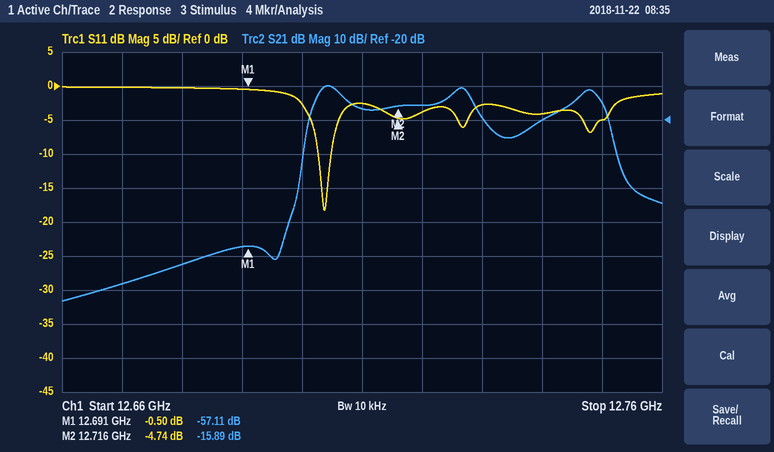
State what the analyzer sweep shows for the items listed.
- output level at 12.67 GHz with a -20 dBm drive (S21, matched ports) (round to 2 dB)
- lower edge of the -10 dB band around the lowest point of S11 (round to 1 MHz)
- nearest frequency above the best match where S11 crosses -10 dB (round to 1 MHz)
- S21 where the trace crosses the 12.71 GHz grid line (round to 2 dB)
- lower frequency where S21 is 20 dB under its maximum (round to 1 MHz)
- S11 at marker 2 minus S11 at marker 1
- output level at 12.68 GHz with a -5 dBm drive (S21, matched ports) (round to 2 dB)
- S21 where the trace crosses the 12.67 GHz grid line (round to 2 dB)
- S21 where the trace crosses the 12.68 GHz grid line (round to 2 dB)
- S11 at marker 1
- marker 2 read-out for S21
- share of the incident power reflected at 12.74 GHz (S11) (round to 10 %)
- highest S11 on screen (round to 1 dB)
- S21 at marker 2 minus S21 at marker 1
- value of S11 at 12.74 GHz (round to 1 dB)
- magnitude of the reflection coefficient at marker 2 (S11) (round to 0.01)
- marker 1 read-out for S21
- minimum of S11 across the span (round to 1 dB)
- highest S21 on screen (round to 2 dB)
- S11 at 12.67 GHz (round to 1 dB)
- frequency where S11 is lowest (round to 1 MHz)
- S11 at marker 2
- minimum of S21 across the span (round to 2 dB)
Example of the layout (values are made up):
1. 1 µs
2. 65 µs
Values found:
1. -88 dBm
2. 12.703 GHz
3. 12.705 GHz
4. -16 dB
5. 12.700 GHz
6. -4.24 dB
7. -68 dBm
8. -68 dB
9. -62 dB
10. -0.50 dB
11. -15.89 dB
12. 40 %
13. 0 dB
14. 41.22 dB
15. -4 dB
16. 0.58
17. -57.11 dB
18. -18 dB
19. -10 dB
20. 0 dB
21. 12.704 GHz
22. -4.74 dB
23. -74 dB
